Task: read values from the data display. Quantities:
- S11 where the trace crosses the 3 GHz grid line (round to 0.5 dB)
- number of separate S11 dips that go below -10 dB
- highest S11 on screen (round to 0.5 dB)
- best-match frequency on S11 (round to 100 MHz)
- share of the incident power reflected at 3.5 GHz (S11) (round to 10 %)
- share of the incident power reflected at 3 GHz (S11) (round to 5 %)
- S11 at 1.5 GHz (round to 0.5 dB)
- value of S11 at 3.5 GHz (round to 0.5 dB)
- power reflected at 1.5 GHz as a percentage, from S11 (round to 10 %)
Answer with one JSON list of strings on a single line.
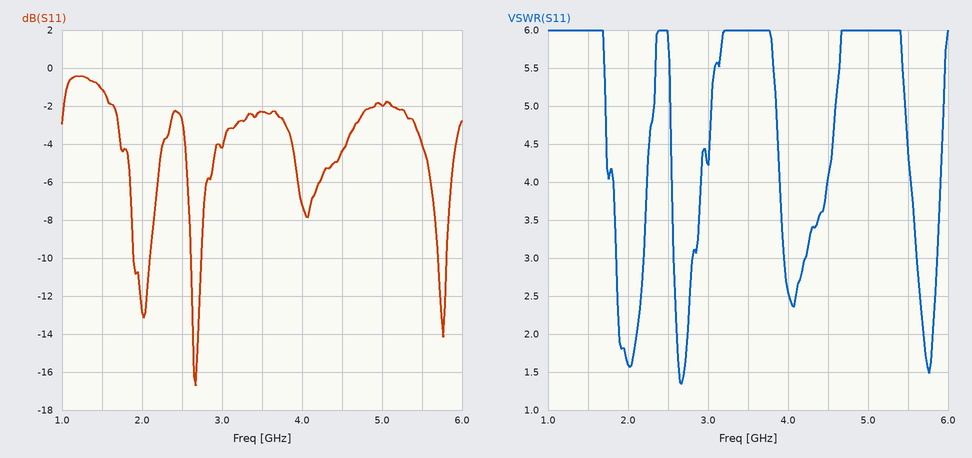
["-4.0 dB", "3", "-0.5 dB", "2.7 GHz", "60 %", "40 %", "-1.0 dB", "-2.5 dB", "80 %"]
